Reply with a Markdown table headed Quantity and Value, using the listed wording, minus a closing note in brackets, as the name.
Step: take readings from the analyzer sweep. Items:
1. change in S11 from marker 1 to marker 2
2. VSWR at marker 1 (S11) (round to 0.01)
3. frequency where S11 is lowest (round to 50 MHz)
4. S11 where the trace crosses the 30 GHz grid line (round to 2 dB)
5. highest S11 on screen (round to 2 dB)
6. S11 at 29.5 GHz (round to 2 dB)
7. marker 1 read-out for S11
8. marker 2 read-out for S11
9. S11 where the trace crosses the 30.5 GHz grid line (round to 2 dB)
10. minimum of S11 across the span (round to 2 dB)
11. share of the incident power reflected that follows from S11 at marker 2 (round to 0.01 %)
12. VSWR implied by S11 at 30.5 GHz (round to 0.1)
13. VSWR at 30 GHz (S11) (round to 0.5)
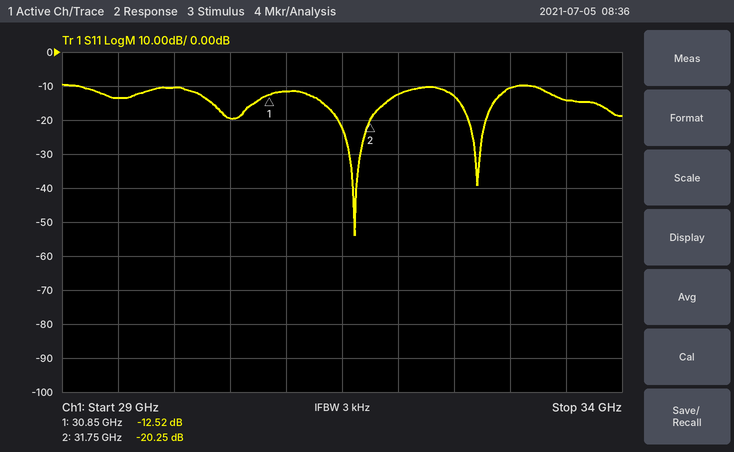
| Quantity | Value |
|---|---|
| change in S11 from marker 1 to marker 2 | -7.73 dB |
| VSWR at marker 1 (S11) | 1.62 |
| frequency where S11 is lowest | 31.60 GHz |
| S11 where the trace crosses the 30 GHz grid line | -10 dB |
| highest S11 on screen | -10 dB |
| S11 at 29.5 GHz | -14 dB |
| marker 1 read-out for S11 | -12.52 dB |
| marker 2 read-out for S11 | -20.25 dB |
| S11 where the trace crosses the 30.5 GHz grid line | -20 dB |
| minimum of S11 across the span | -54 dB |
| share of the incident power reflected that follows from S11 at marker 2 | 0.94 % |
| VSWR implied by S11 at 30.5 GHz | 1.2 |
| VSWR at 30 GHz (S11) | 2.0 |
